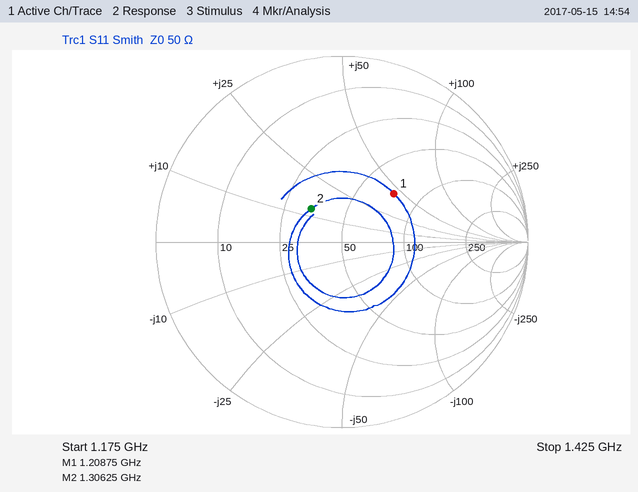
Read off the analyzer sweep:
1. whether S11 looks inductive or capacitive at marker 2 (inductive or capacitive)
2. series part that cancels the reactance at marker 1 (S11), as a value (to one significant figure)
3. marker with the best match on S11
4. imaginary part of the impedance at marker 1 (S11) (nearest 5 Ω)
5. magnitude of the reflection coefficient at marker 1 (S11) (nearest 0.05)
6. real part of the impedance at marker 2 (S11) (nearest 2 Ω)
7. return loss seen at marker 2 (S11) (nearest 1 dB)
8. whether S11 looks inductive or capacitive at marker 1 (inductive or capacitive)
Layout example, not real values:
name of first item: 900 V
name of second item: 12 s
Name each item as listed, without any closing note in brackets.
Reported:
whether S11 looks inductive or capacitive at marker 2: inductive
series part that cancels the reactance at marker 1 (S11), as a value: 3 pF
marker with the best match on S11: marker 2
imaginary part of the impedance at marker 1 (S11): +45 Ω
magnitude of the reflection coefficient at marker 1 (S11): 0.40
real part of the impedance at marker 2 (S11): 34 Ω
return loss seen at marker 2 (S11): 12 dB
whether S11 looks inductive or capacitive at marker 1: inductive
